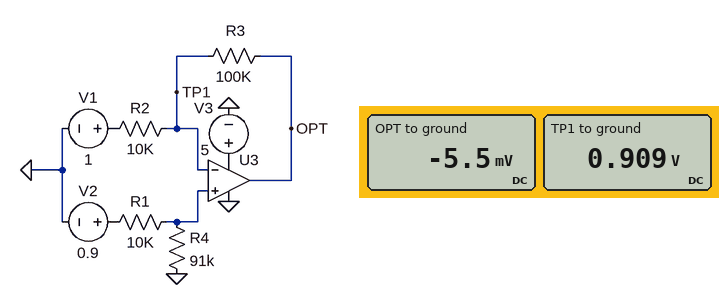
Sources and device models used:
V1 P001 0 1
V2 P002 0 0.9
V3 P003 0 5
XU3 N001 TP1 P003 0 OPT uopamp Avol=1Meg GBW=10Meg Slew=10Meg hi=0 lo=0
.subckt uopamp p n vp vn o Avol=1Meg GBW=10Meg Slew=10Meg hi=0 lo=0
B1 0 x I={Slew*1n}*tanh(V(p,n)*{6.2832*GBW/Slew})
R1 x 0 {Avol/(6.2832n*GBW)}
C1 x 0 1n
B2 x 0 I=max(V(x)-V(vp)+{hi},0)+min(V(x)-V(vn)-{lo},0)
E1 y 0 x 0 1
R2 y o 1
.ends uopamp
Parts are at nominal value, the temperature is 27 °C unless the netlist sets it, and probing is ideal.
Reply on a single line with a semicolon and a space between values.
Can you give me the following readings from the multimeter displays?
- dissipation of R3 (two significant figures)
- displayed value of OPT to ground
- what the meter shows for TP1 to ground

8.4 µW; -5.5 mV; 0.909 V
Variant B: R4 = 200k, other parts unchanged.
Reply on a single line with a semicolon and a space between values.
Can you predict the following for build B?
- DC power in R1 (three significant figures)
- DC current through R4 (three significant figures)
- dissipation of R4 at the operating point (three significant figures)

184 nW; 4.29 µA; 3.67 µW
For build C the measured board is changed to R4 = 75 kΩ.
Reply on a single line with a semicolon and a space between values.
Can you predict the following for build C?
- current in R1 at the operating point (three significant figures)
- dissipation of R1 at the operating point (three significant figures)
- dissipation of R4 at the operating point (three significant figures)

10.6 µA; 1.12 µW; 8.41 µW
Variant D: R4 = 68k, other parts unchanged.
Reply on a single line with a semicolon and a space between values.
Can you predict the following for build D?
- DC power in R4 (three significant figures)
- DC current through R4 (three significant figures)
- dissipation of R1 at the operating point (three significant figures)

9.05 µW; 11.5 µA; 1.33 µW
